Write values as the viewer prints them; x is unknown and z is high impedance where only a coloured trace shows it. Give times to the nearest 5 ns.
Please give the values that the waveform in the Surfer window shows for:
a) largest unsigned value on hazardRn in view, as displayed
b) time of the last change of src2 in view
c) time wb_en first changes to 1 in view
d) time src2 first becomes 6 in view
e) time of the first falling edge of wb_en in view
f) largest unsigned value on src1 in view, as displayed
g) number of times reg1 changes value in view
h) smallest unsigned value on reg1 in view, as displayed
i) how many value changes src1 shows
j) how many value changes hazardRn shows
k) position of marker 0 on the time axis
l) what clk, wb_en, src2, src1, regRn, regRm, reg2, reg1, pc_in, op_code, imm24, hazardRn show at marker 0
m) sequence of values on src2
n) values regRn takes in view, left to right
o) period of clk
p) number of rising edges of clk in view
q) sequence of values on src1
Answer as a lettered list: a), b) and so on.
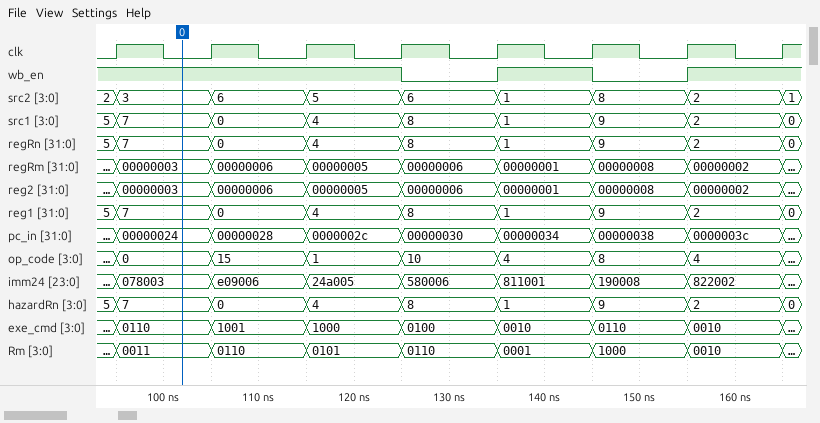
a) 9
b) 165 ns
c) 135 ns
d) 105 ns
e) 125 ns
f) 9
g) 8
h) 0
i) 8
j) 8
k) 100 ns
l) clk=0, wb_en=1, src2=3, src1=7, regRn=7, regRm=00000003, reg2=00000003, reg1=7, pc_in=00000024, op_code=0, imm24=078003, hazardRn=7
m) 2, 3, 6, 5, 6, 1, 8, 2, 1
n) 5, 7, 0, 4, 8, 1, 9, 2, 0
o) 10 ns
p) 8
q) 5, 7, 0, 4, 8, 1, 9, 2, 0
